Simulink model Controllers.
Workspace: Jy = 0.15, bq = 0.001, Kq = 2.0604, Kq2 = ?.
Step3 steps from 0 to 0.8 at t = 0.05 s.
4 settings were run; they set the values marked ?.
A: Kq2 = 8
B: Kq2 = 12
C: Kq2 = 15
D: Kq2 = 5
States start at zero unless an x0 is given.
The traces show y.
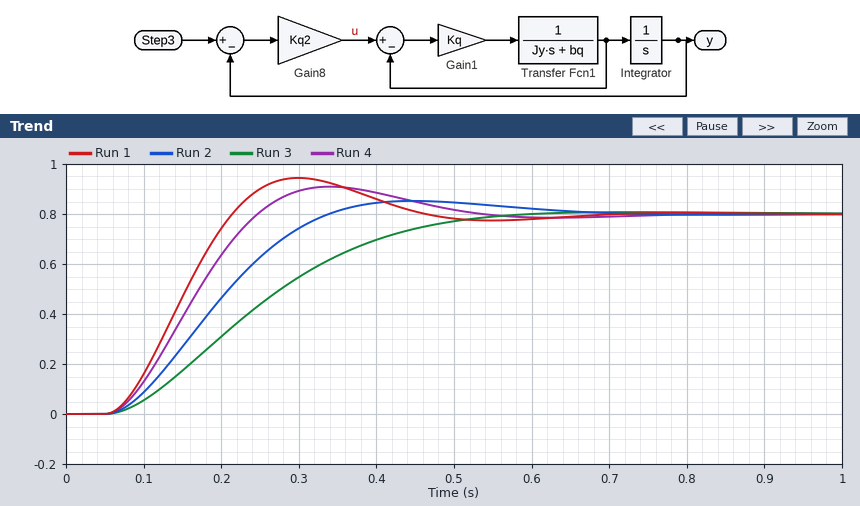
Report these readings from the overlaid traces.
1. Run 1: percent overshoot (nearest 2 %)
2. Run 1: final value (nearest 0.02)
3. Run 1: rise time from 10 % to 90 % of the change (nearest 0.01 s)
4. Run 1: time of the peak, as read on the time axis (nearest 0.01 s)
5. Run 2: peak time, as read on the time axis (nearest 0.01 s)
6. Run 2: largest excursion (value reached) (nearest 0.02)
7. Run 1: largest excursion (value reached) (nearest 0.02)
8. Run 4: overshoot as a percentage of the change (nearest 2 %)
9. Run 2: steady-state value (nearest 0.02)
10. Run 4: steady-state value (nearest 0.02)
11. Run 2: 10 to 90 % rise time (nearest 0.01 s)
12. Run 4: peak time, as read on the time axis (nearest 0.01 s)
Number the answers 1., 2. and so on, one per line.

1. 18 %
2. 0.80
3. 0.11 s
4. 0.30 s
5. 0.45 s
6. 0.86
7. 0.94
8. 14 %
9. 0.80
10. 0.80
11. 0.19 s
12. 0.34 s
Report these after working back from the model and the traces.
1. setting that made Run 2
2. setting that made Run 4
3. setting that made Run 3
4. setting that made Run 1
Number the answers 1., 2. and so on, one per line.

1. A
2. B
3. D
4. C
